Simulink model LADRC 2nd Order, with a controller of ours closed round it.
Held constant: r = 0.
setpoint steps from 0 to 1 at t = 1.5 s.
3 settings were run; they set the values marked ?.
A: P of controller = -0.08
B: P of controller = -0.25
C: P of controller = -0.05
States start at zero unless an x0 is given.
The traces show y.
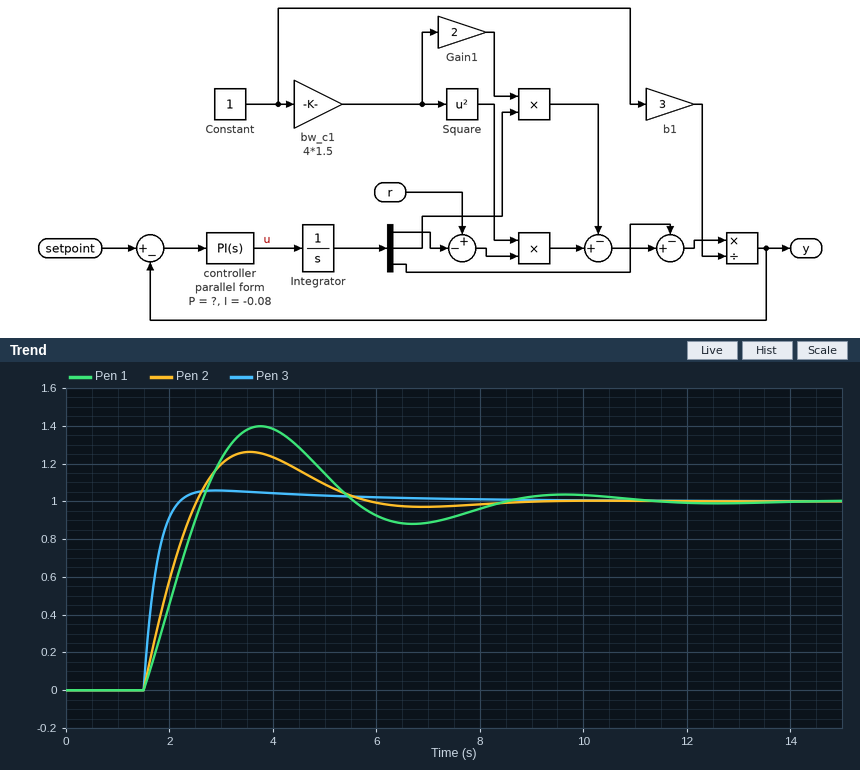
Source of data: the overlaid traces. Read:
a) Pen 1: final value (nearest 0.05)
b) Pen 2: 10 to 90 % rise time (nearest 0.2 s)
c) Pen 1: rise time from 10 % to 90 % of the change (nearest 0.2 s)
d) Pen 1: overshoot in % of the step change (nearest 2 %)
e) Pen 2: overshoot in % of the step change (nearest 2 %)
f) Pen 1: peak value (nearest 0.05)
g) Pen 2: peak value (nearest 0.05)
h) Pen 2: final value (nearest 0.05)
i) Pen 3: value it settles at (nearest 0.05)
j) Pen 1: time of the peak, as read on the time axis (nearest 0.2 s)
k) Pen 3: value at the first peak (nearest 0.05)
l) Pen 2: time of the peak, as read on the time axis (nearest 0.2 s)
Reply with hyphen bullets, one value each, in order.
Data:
- 1.00
- 0.8 s
- 0.8 s
- 40 %
- 26 %
- 1.40
- 1.25
- 1.00
- 1.00
- 3.8 s
- 1.05
- 3.6 s
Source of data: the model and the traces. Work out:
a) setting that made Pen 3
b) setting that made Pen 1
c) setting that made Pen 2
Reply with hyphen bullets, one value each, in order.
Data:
- B
- C
- A
